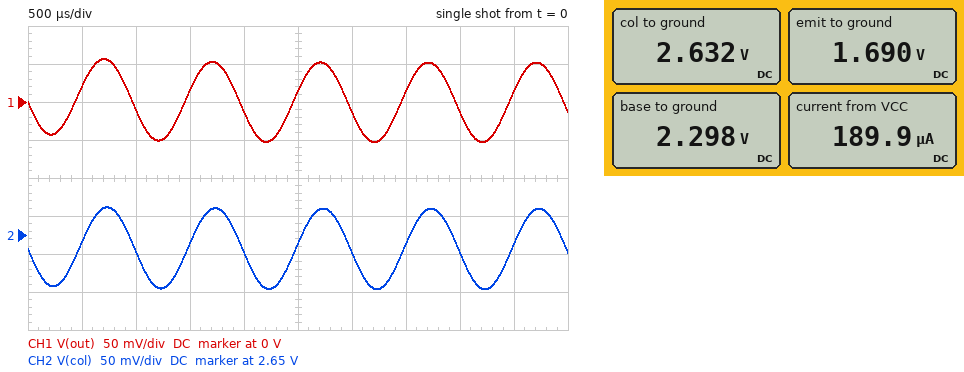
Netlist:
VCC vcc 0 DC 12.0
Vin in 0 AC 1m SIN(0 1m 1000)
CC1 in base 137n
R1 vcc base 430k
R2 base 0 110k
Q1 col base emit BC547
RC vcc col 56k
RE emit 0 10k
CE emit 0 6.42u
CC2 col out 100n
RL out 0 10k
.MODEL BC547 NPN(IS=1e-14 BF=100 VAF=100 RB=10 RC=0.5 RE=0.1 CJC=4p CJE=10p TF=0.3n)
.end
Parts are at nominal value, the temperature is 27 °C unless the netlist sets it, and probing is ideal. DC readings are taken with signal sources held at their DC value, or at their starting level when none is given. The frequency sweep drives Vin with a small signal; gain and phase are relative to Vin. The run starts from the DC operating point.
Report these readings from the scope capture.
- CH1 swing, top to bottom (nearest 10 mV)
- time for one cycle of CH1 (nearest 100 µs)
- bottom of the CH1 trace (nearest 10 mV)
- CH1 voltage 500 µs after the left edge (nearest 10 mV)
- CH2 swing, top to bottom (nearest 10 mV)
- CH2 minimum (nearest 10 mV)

110 mV
1.0 ms
-50 mV
20 mV
110 mV
2.58 V
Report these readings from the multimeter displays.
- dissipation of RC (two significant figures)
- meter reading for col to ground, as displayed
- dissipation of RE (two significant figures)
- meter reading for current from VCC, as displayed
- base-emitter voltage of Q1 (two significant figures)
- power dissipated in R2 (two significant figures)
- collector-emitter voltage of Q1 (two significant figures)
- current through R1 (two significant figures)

1.6 mW
2.632 V
290 µW
189.9 µA
610 mV
48 µW
940 mV
23 µA
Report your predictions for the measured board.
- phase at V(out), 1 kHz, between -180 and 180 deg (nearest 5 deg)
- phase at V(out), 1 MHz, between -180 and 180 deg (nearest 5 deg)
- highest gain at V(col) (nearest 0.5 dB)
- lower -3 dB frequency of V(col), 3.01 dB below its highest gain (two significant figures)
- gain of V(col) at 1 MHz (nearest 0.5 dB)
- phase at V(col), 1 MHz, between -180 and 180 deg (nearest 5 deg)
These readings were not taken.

-165 deg
170 deg
34.5 dB
110 Hz
34.5 dB
170 deg
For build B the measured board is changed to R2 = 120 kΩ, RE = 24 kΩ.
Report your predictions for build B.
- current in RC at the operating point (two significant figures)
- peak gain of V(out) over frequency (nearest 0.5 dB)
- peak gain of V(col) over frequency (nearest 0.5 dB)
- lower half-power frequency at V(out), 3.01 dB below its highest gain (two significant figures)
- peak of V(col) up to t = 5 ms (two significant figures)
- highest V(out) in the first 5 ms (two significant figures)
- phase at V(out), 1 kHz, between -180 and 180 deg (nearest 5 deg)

81 µA
28.5 dB
30.0 dB
120 Hz
7.5 V
28 mV
-170 deg
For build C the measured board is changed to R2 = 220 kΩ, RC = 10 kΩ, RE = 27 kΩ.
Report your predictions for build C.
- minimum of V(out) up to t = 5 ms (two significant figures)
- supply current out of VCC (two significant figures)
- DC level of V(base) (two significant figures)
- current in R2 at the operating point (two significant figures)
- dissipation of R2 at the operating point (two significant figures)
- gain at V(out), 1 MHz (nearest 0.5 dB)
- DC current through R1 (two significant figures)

-23 mV
140 µA
3.9 V
18 µA
69 µW
27.5 dB
19 µA
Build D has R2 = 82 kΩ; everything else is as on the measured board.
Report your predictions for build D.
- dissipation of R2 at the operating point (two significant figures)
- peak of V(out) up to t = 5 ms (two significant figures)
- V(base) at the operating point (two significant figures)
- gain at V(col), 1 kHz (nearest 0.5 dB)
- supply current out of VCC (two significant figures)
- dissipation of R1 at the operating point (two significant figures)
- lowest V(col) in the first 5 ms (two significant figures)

41 µW
42 mV
1.8 V
32.0 dB
150 µA
240 µW
5.1 V
